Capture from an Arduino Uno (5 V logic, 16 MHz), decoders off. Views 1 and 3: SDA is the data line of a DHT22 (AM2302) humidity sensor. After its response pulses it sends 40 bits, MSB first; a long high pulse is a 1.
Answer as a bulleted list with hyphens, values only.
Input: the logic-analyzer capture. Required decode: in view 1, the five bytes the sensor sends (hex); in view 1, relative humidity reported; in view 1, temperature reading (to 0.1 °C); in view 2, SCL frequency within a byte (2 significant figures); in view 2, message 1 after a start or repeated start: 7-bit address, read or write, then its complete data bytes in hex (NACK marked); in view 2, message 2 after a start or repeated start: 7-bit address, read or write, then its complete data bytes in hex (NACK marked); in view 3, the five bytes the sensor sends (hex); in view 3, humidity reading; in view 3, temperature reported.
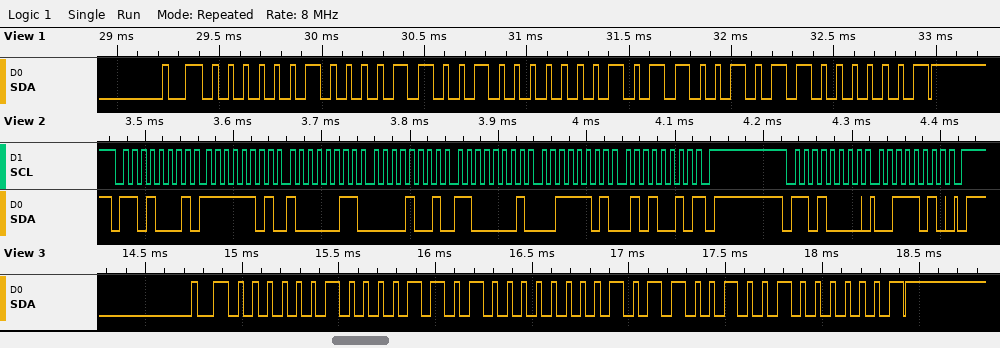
- 02 19 01 65 81
- 53.7 %
- 35.7 °C
- 100 kHz
- 0x68 read: FD 83 09 C1 3D 52 NACK
- 0x68 write: 3A
- 02 1A 01 64 81
- 53.8 %
- 35.6 °C
